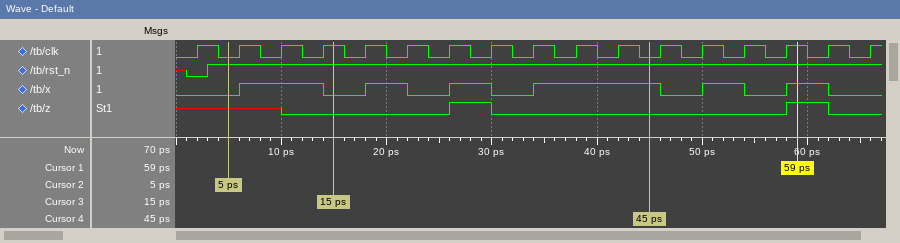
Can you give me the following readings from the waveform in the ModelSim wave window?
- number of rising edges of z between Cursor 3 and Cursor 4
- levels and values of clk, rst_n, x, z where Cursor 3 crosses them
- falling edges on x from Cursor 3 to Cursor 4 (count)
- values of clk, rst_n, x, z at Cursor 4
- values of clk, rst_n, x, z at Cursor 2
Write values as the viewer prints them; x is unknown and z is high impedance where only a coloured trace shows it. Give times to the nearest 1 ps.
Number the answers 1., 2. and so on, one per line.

1. 1
2. clk=1, rst_n=1, x=0, z=0
3. 2
4. clk=0, rst_n=1, x=1, z=0
5. clk=0, rst_n=1, x=0, z=x
